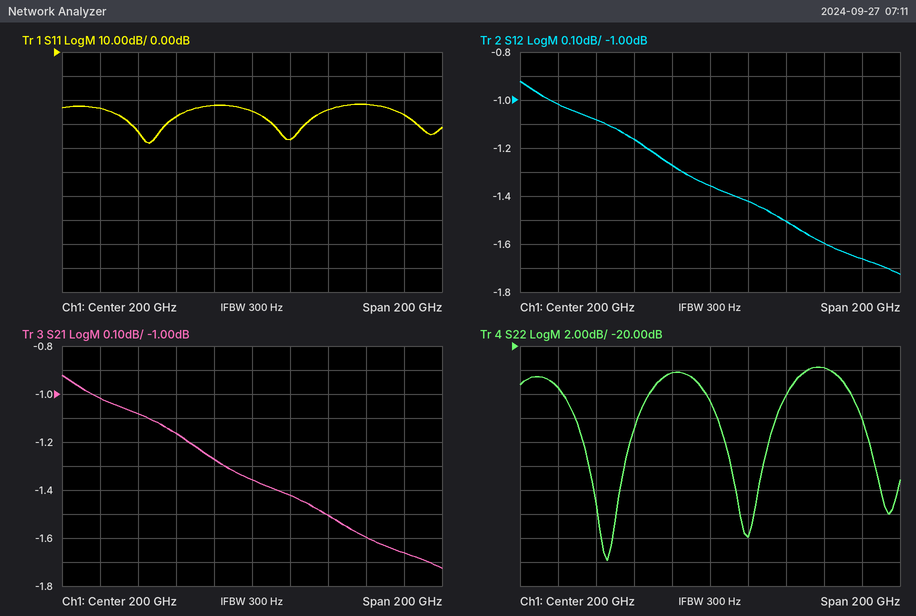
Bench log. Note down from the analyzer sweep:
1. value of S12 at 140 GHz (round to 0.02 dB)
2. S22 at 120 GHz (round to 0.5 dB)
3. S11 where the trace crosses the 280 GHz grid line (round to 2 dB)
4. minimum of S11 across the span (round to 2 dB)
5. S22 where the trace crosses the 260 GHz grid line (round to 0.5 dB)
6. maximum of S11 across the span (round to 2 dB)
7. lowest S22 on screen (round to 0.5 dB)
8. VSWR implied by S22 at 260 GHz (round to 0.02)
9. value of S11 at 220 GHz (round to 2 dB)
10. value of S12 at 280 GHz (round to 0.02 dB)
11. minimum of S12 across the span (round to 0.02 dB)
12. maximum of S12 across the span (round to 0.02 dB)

-1.08 dB
-23.5 dB
-26 dB
-38 dB
-22.0 dB
-22 dB
-38.0 dB
1.18
-36 dB
-1.66 dB
-1.72 dB
-0.92 dB
